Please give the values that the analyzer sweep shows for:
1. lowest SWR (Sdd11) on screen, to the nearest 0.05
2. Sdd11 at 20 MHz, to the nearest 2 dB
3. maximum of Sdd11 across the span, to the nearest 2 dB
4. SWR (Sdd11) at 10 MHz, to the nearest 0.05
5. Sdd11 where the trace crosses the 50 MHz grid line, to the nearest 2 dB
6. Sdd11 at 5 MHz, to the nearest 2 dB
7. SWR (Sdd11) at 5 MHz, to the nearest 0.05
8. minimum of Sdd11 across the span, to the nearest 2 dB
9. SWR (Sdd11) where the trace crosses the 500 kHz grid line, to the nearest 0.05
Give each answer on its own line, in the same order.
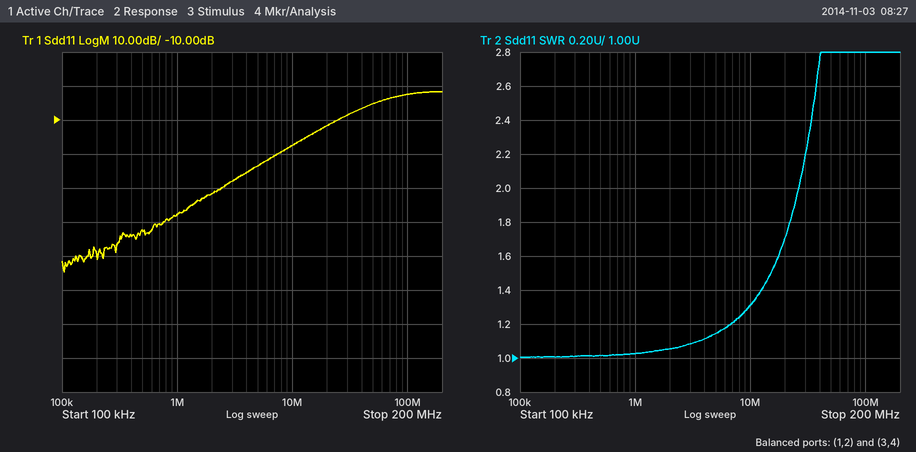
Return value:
1.00
-12 dB
-2 dB
1.30
-6 dB
-24 dB
1.15
-54 dB
1.00
